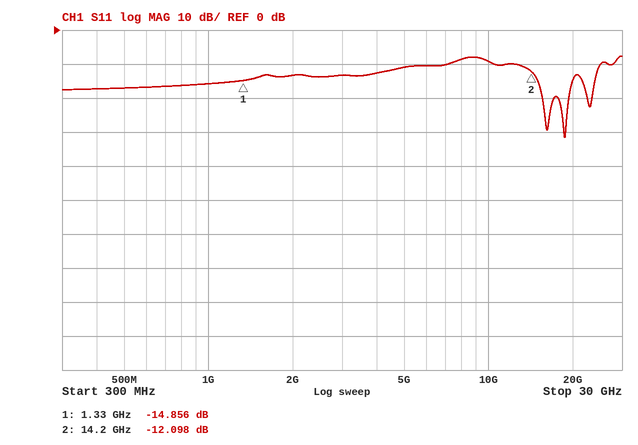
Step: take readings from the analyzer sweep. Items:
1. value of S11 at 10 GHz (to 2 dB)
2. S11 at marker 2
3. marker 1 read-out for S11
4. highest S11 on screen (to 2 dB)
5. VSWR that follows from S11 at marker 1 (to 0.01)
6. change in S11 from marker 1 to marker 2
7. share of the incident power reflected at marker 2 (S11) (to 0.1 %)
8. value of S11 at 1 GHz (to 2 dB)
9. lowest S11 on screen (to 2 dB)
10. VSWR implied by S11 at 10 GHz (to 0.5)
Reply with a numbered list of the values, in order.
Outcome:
1. -10 dB
2. -12.098 dB
3. -14.856 dB
4. -8 dB
5. 1.44
6. 2.758 dB
7. 6.2 %
8. -16 dB
9. -32 dB
10. 2.0
